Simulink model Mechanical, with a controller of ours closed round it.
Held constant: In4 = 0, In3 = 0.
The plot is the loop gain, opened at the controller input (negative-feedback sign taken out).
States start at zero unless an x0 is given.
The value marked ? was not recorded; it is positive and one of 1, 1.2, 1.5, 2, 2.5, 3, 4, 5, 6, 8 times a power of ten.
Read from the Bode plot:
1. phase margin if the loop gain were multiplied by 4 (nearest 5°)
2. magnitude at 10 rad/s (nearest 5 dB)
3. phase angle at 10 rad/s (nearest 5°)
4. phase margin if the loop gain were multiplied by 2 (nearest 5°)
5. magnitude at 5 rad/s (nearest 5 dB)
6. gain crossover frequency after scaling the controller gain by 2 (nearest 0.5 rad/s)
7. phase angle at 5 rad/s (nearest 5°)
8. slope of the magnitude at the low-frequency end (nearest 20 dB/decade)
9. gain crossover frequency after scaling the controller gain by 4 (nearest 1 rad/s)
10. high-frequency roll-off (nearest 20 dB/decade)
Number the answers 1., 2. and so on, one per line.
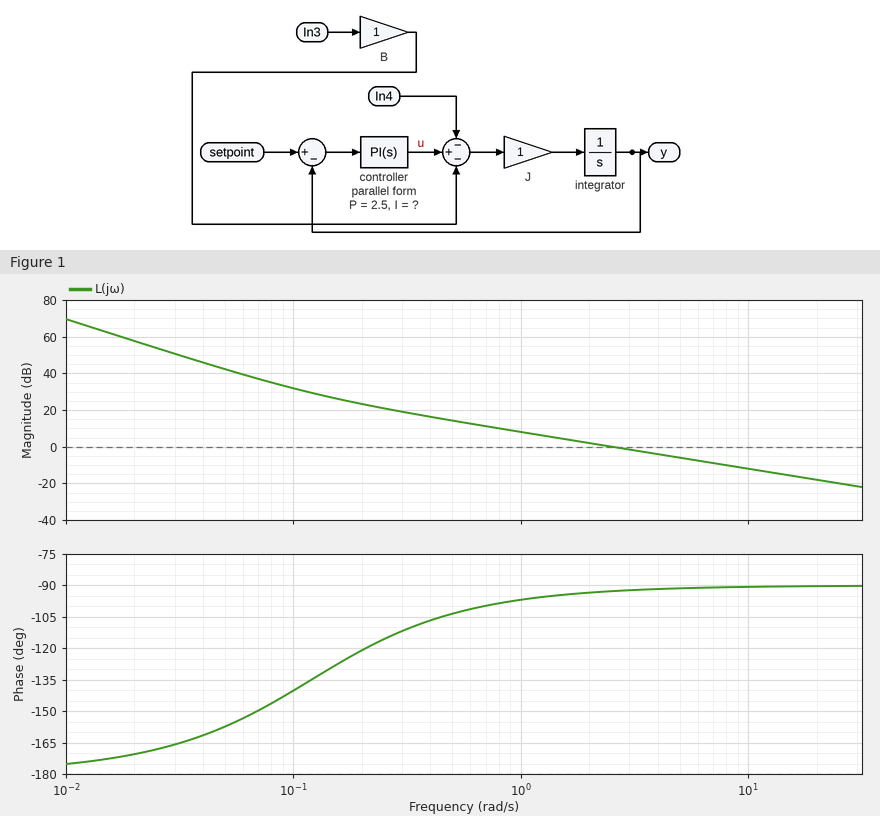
1. 90°
2. -10 dB
3. -90°
4. 90°
5. -5 dB
6. 5.0 rad/s
7. -90°
8. -40 dB/decade
9. 10 rad/s
10. -20 dB/decade
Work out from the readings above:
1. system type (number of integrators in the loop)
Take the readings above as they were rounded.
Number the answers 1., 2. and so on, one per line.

1. 2
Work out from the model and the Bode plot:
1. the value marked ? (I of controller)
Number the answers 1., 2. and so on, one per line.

1. 0.3
